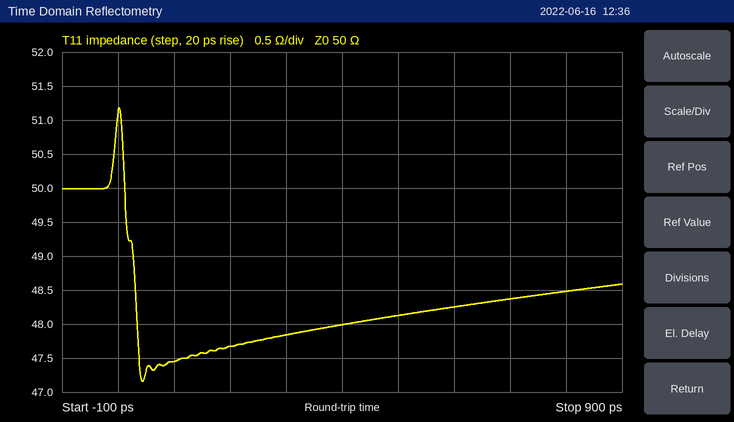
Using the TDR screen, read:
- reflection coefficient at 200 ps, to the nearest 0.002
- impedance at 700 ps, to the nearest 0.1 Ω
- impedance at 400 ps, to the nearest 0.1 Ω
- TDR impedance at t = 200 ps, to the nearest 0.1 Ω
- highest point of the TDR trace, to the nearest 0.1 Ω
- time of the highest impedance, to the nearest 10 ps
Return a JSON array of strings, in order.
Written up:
["-0.024", "48.4 Ω", "48.0 Ω", "47.7 Ω", "51.2 Ω", "0 ps"]
